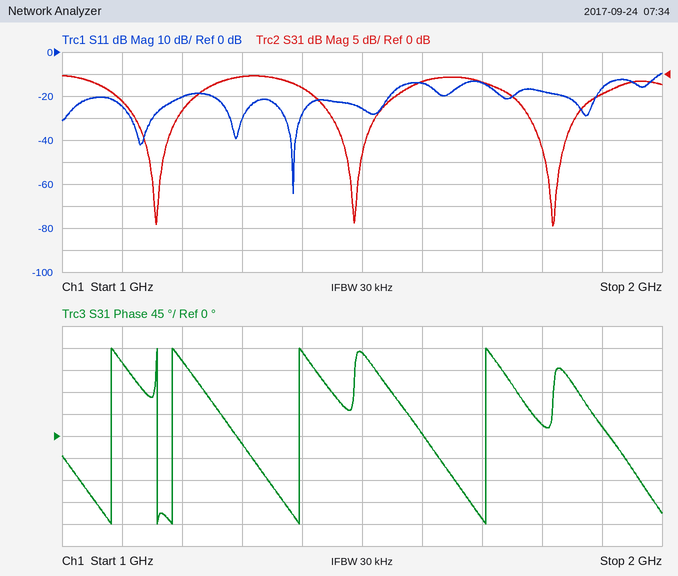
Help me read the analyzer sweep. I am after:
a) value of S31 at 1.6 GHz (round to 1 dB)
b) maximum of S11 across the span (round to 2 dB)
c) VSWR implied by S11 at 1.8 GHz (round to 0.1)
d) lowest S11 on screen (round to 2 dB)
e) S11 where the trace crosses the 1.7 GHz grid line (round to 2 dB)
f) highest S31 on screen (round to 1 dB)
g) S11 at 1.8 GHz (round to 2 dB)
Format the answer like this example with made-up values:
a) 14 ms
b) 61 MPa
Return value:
a) -2 dB
b) -10 dB
c) 1.3
d) -64 dB
e) -14 dB
f) 0 dB
g) -18 dB
